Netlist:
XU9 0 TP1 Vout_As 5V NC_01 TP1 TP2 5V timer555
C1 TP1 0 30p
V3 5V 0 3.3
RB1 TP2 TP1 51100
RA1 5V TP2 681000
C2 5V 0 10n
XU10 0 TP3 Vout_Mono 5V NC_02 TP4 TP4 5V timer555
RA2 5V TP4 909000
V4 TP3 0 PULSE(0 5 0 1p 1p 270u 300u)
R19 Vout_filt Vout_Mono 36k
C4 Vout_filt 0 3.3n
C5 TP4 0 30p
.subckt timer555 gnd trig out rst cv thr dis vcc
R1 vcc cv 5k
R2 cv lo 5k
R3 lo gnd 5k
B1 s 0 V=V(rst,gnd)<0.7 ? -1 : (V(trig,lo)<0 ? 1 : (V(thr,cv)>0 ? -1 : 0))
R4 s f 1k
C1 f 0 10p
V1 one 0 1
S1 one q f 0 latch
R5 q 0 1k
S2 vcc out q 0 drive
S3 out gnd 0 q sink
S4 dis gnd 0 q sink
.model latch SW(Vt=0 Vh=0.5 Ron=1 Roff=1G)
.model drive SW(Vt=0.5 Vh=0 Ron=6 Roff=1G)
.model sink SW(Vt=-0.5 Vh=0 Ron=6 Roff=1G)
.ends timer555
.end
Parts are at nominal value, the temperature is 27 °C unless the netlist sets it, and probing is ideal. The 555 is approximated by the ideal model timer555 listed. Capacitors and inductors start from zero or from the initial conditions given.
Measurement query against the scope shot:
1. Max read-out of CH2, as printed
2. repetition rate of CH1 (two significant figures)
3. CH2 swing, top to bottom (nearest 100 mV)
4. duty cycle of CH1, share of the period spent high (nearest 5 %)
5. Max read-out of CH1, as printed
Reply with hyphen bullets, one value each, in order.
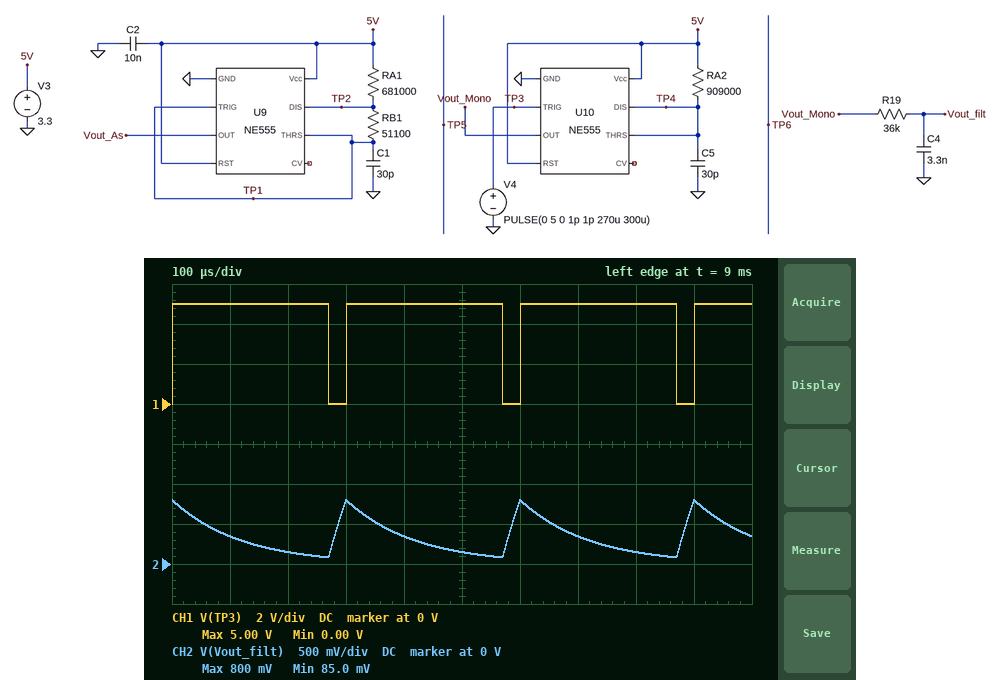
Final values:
- 800 mV
- 3.3 kHz
- 700 mV
- 90 %
- 5.00 V
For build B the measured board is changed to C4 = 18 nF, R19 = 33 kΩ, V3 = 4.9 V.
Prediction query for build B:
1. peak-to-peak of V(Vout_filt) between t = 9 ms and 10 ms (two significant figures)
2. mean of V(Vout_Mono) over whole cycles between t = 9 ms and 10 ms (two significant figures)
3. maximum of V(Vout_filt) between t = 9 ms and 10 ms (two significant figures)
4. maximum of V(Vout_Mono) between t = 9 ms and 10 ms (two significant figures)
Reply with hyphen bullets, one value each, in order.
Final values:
- 220 mV
- 490 mV
- 610 mV
- 4.9 V
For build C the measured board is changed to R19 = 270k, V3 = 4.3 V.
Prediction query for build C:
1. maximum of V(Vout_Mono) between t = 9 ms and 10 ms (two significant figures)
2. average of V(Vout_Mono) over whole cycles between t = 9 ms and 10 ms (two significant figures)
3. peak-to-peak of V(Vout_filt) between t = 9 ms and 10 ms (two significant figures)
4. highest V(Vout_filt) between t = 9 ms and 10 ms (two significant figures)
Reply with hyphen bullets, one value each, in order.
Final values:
- 4.3 V
- 430 mV
- 130 mV
- 500 mV
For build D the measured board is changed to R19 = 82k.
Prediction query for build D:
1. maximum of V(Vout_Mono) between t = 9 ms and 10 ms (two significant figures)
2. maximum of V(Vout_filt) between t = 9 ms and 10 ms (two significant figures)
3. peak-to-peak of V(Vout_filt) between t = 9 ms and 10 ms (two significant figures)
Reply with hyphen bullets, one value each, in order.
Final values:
- 3.3 V
- 520 mV
- 330 mV
